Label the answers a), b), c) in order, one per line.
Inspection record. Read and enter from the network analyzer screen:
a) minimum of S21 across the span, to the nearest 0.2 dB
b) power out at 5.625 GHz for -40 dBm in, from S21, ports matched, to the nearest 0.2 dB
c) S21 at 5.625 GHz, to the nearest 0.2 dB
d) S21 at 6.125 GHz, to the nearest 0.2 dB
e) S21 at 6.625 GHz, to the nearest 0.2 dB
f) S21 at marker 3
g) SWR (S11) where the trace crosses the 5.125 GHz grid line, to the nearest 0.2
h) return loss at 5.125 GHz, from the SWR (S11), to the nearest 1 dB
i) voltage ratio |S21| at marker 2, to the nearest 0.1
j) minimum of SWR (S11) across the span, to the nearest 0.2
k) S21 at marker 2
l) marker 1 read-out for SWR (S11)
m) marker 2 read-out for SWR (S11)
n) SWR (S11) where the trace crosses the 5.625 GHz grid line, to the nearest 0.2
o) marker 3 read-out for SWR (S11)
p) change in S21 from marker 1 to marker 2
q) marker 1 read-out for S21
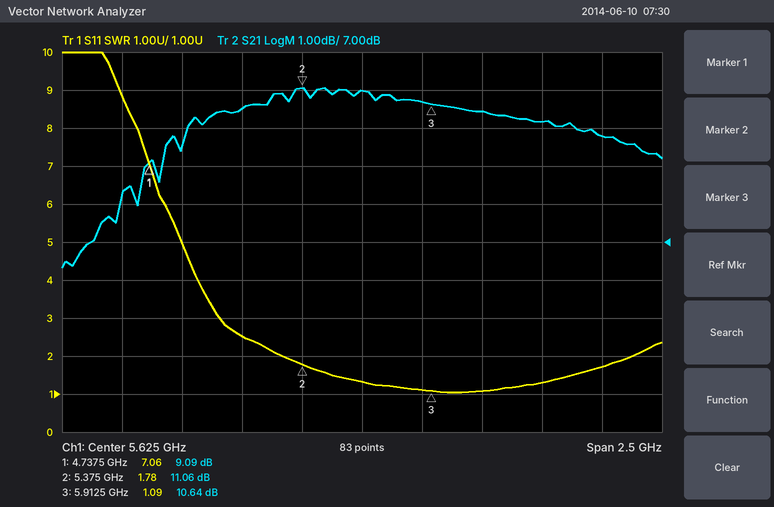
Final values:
a) 6.4 dB
b) -29.0 dBm
c) 11.0 dB
d) 10.4 dB
e) 9.8 dB
f) 10.64 dB
g) 2.6
h) 7 dB
i) 3.6
j) 1.0
k) 11.06 dB
l) 7.06
m) 1.78
n) 1.4
o) 1.09
p) 1.97 dB
q) 9.09 dB
